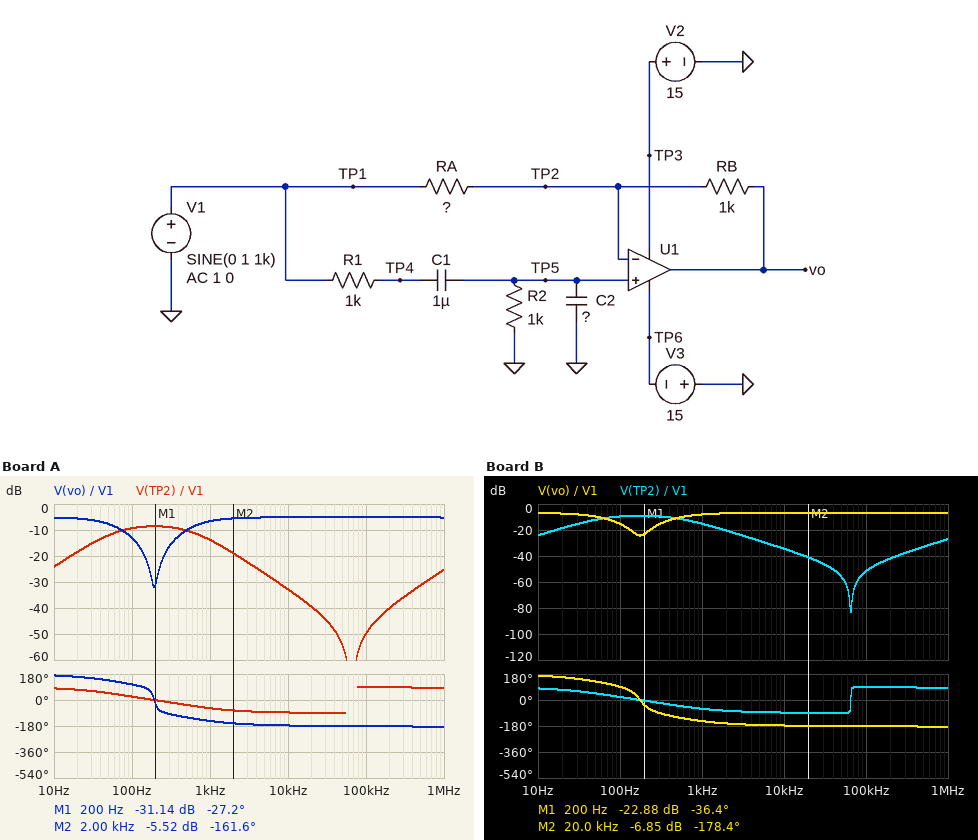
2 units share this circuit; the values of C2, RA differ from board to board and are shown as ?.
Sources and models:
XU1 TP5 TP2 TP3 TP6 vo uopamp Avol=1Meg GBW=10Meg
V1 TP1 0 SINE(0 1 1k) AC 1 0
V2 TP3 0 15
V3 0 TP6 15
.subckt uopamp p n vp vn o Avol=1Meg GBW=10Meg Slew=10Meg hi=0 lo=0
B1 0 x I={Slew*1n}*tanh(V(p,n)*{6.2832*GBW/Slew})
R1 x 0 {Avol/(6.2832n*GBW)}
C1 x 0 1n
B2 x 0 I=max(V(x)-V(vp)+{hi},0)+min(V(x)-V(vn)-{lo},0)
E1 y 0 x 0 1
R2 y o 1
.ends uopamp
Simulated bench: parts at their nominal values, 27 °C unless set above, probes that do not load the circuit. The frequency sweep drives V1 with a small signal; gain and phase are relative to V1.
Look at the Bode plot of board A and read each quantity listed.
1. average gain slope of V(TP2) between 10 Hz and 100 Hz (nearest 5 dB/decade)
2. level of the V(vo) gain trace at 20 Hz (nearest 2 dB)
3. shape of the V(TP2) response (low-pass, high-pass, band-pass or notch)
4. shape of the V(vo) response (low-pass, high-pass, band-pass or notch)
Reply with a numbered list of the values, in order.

1. 15 dB/decade
2. -6 dB
3. band-pass
4. notch
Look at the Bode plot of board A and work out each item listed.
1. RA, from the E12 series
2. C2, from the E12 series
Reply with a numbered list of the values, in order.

1. 1.8 kΩ
2. 680 nF
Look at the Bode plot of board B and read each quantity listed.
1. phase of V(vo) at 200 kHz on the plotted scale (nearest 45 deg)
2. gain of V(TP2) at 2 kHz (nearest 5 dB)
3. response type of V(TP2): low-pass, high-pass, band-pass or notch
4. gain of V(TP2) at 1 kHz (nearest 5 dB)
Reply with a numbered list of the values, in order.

1. -180 deg
2. -20 dB
3. band-pass
4. -15 dB
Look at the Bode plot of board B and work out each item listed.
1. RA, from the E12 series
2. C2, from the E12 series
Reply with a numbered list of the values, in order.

1. 2.2 kΩ
2. 820 nF
